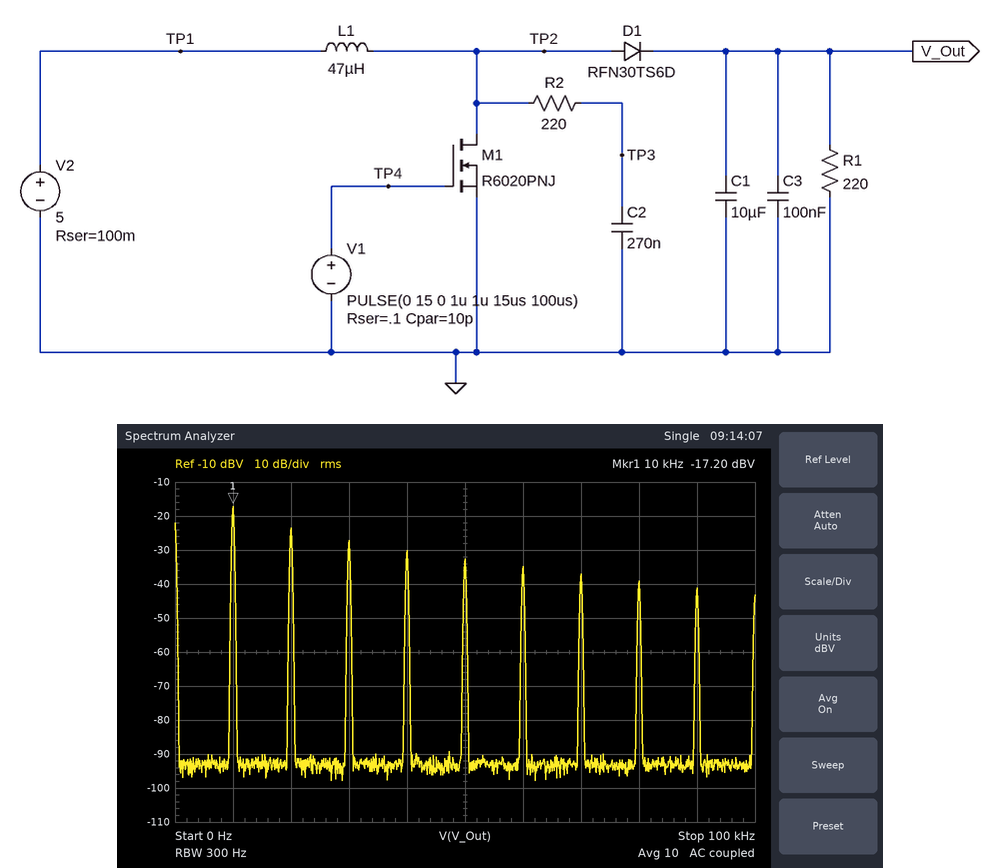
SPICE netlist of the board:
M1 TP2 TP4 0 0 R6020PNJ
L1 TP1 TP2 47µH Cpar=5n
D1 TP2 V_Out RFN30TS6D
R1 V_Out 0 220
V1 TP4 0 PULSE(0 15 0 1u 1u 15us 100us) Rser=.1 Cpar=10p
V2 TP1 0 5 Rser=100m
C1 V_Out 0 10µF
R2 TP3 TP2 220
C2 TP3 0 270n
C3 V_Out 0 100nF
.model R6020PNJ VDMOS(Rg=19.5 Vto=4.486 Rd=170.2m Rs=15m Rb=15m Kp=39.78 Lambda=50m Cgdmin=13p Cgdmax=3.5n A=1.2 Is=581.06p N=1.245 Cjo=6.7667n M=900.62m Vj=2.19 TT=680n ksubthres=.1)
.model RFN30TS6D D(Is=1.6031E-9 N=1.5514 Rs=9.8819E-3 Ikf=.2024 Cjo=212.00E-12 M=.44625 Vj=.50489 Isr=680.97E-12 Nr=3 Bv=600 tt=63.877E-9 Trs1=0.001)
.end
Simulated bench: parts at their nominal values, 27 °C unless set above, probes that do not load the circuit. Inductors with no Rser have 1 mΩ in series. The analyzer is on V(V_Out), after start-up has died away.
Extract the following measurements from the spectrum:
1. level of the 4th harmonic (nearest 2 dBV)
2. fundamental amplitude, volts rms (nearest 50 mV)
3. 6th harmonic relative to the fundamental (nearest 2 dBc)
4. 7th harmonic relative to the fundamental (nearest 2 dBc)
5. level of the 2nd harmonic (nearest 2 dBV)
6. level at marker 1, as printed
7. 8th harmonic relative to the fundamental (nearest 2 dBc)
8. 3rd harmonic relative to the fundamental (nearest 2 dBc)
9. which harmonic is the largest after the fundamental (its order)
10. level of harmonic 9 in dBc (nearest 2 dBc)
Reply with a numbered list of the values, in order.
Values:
1. -30 dBV
2. 150 mV
3. -18 dBc
4. -20 dBc
5. -24 dBV
6. -17.20 dBV
7. -22 dBc
8. -10 dBc
9. 2
10. -24 dBc
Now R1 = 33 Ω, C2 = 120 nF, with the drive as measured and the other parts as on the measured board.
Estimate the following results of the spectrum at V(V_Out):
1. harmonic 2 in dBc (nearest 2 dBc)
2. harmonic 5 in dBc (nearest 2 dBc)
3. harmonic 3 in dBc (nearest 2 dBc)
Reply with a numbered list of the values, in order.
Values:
1. -8 dBc
2. -26 dBc
3. -14 dBc
